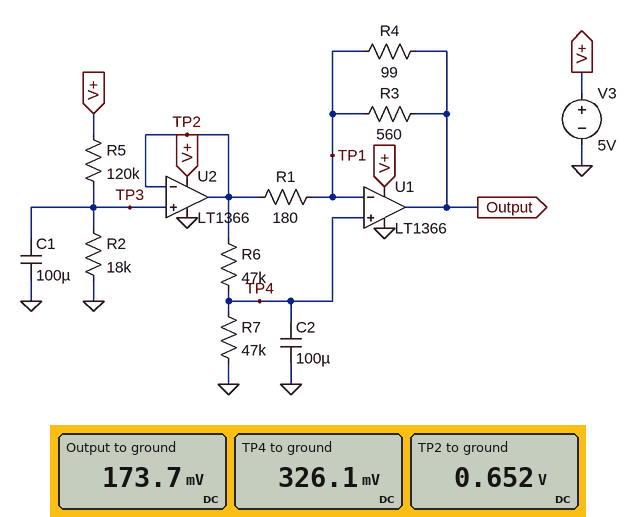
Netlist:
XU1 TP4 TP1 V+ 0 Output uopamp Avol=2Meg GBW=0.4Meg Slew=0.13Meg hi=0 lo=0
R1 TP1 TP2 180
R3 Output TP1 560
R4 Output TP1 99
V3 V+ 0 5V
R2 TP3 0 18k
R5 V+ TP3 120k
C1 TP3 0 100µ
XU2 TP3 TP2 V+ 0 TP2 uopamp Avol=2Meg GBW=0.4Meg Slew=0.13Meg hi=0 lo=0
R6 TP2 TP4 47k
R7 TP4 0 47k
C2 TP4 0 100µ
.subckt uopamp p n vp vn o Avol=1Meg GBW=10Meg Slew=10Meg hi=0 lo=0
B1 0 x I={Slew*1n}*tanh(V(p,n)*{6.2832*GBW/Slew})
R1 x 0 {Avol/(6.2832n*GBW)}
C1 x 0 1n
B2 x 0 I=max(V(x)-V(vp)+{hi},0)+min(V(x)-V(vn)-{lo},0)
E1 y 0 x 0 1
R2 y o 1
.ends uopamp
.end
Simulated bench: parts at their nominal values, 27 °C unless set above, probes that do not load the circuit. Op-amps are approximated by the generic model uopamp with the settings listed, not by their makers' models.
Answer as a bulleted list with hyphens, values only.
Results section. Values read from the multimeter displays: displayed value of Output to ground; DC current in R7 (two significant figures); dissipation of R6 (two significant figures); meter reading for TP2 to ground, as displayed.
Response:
- 173.7 mV
- 6.9 µA
- 2.3 µW
- 0.652 V
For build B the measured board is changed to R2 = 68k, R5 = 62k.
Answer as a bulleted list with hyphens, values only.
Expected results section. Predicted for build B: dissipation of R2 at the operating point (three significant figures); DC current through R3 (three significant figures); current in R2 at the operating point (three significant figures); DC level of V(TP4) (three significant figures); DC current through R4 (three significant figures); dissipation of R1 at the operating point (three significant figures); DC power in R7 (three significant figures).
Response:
- 101 µW
- 1.09 mA
- 38.5 µA
- 1.31 V
- 6.17 mA
- 9.50 mW
- 36.4 µW
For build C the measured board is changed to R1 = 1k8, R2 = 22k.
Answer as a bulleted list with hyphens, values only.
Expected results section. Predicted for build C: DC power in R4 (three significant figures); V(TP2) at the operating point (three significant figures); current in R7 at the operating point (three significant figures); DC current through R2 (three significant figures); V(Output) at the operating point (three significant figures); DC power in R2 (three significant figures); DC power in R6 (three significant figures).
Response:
- 3.31 µW
- 775 mV
- 8.24 µA
- 35.2 µA
- 369 mV
- 27.3 µW
- 3.19 µW
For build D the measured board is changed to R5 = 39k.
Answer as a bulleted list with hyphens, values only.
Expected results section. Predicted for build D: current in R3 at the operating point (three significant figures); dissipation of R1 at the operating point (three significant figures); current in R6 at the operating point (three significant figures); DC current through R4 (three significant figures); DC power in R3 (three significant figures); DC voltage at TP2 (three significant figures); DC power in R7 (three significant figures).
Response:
- 659 µA
- 3.46 mW
- 16.8 µA
- 3.73 mA
- 243 µW
- 1.58 V
- 13.3 µW
